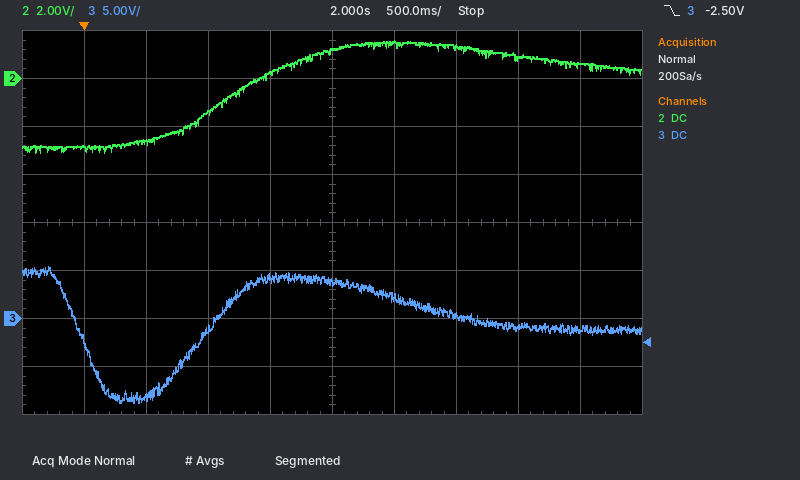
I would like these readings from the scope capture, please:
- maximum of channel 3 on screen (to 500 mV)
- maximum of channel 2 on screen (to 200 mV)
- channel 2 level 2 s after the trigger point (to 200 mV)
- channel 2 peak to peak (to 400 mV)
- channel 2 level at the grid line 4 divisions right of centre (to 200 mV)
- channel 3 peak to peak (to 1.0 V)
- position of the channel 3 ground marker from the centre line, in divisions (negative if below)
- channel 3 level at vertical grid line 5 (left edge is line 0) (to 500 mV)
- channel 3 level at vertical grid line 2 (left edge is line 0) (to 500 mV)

5.5 V
1.6 V
1.2 V
4.8 V
600 mV
14.0 V
-2.0 div
4.0 V
-8.0 V
